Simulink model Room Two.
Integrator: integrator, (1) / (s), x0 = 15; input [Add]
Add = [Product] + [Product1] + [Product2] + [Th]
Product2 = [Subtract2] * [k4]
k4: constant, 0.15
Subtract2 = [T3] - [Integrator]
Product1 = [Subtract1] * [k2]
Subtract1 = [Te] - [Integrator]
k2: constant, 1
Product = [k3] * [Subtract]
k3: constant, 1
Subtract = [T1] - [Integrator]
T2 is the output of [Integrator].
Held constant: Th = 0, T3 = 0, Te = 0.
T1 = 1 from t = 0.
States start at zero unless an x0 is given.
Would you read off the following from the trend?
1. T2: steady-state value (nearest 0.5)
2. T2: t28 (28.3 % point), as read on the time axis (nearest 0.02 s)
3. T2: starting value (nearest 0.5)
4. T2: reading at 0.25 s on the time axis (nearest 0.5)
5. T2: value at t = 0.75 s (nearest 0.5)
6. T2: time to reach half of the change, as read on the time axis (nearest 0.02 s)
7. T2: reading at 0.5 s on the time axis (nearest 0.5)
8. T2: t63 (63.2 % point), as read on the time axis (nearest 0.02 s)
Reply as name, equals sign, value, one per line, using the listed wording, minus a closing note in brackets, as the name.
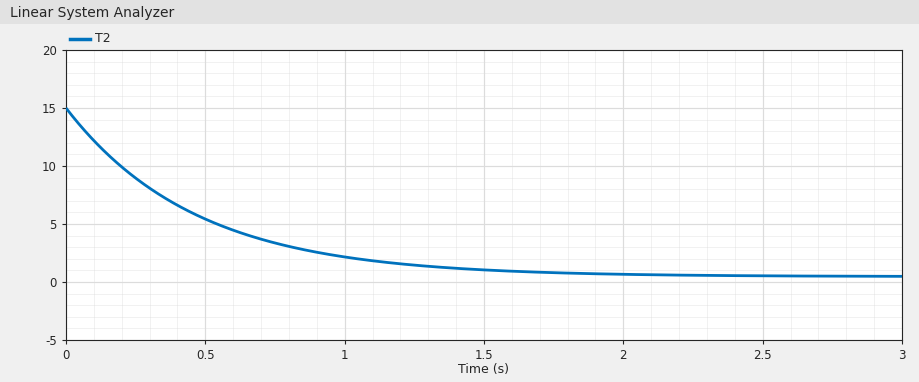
T2: steady-state value = 0.5
T2: t28 (28.3 % point), as read on the time axis = 0.16 s
T2: starting value = 15.0
T2: reading at 0.25 s on the time axis = 9.0
T2: value at t = 0.75 s = 3.5
T2: time to reach half of the change, as read on the time axis = 0.32 s
T2: reading at 0.5 s on the time axis = 5.5
T2: t63 (63.2 % point), as read on the time axis = 0.46 s
